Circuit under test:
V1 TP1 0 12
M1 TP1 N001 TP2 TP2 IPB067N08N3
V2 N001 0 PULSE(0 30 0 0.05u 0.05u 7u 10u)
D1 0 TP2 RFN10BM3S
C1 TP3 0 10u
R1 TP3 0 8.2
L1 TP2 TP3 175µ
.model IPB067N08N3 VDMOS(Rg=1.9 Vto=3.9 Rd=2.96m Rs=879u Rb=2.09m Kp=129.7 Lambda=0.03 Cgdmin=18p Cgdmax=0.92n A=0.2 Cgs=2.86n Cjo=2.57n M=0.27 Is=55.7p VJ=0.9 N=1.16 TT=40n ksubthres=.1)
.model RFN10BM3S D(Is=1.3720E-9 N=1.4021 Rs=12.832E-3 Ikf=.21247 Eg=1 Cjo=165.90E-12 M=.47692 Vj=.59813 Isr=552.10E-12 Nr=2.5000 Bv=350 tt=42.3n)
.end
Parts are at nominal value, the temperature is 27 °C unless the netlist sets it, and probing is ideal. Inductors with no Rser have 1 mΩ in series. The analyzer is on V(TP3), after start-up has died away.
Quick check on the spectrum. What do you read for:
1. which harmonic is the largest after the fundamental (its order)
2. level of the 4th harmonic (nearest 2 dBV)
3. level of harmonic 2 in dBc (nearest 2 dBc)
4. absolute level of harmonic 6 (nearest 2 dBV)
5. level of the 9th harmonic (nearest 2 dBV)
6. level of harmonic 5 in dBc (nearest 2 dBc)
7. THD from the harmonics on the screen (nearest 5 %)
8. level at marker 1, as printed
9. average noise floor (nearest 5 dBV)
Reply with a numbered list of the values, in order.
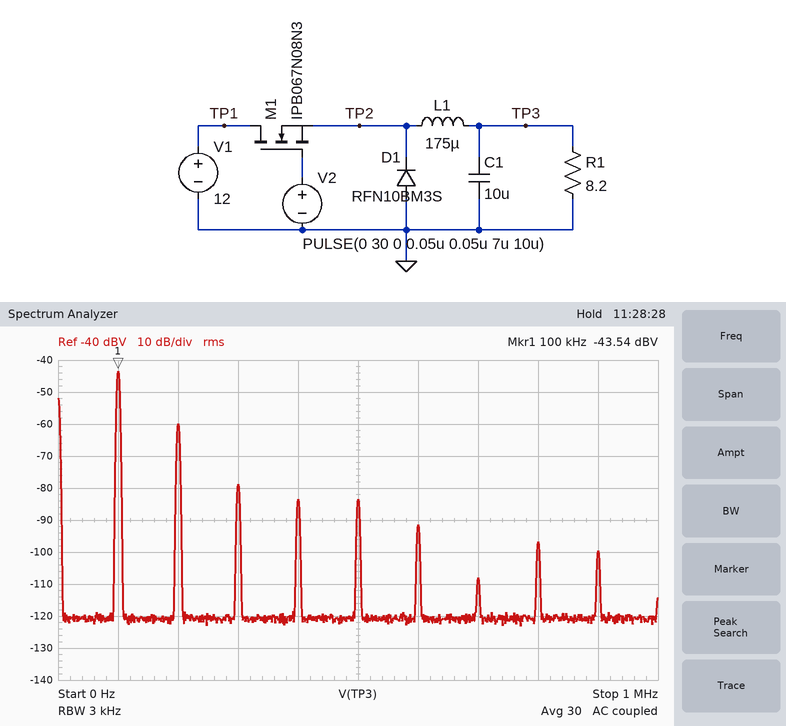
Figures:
1. 2
2. -84 dBV
3. -16 dBc
4. -92 dBV
5. -100 dBV
6. -40 dBc
7. 15 %
8. -43.54 dBV
9. -120 dBV
